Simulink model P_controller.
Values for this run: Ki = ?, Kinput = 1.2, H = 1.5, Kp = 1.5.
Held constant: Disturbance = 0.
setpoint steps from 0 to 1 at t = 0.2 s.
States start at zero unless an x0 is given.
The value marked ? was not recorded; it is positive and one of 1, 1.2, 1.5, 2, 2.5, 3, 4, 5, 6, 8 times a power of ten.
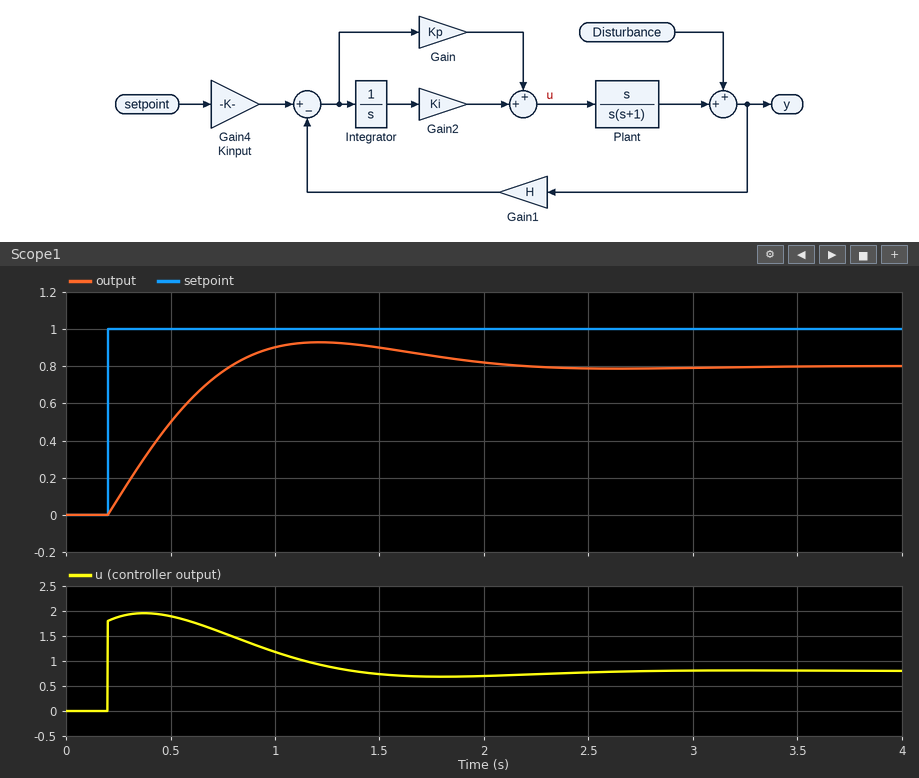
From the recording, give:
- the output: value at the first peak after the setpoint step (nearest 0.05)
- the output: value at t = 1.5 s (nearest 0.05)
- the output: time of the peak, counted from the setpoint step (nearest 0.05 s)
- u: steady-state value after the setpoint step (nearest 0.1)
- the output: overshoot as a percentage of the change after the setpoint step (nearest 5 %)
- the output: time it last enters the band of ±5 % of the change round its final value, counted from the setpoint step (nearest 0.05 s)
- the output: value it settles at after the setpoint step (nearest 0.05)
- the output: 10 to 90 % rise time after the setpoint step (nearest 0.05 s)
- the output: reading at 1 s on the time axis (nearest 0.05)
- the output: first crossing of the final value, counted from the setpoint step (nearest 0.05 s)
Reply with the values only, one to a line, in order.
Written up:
0.95
0.90
1.00 s
0.8
15 %
1.65 s
0.80
0.45 s
0.90
0.60 s
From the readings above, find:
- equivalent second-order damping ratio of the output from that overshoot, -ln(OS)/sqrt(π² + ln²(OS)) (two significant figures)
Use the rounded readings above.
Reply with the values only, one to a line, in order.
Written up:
0.52
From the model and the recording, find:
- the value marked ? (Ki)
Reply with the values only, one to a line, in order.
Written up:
5
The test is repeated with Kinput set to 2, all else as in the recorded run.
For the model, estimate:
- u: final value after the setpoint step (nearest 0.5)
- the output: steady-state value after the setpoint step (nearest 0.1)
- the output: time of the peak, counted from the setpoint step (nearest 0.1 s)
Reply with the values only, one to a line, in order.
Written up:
1.5
1.3
1.0 s
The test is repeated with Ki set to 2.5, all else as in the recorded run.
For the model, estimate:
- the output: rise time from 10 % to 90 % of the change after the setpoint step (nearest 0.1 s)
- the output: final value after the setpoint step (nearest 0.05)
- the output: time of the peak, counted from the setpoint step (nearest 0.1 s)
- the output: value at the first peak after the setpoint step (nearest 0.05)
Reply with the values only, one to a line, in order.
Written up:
0.7 s
0.80
1.5 s
0.85
